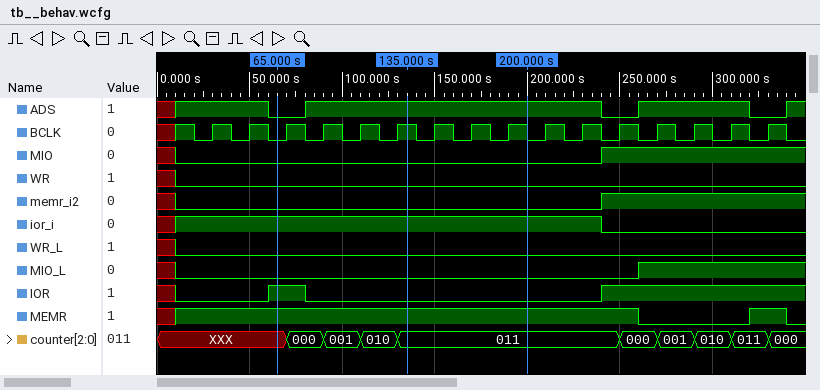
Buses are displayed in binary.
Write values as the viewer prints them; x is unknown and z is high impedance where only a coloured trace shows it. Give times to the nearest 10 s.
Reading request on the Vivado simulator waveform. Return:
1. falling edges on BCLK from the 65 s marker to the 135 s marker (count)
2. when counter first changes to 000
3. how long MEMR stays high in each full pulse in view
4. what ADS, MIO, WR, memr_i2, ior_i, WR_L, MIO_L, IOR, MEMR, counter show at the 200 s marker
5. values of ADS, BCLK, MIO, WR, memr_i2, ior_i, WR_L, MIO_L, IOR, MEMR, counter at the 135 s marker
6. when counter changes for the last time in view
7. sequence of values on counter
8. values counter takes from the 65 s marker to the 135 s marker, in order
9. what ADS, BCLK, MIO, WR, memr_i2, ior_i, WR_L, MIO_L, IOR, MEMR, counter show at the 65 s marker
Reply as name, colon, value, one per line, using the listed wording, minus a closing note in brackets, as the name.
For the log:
falling edges on BCLK from the 65 s marker to the 135 s marker: 3
when counter first changes to 000: 70 s
how long MEMR stays high in each full pulse in view: 20 s
what ADS, MIO, WR, memr_i2, ior_i, WR_L, MIO_L, IOR, MEMR, counter show at the 200 s marker: ADS=1, MIO=0, WR=0, memr_i2=0, ior_i=1, WR_L=0, MIO_L=0, IOR=0, MEMR=1, counter=011
values of ADS, BCLK, MIO, WR, memr_i2, ior_i, WR_L, MIO_L, IOR, MEMR, counter at the 135 s marker: ADS=1, BCLK=1, MIO=0, WR=0, memr_i2=0, ior_i=1, WR_L=0, MIO_L=0, IOR=0, MEMR=1, counter=011
when counter changes for the last time in view: 330 s
sequence of values on counter: XXX, 000, 001, 010, 011, 000, 001, 010, 011, 000
values counter takes from the 65 s marker to the 135 s marker, in order: XXX, 000, 001, 010, 011
what ADS, BCLK, MIO, WR, memr_i2, ior_i, WR_L, MIO_L, IOR, MEMR, counter show at the 65 s marker: ADS=0, BCLK=0, MIO=0, WR=0, memr_i2=0, ior_i=1, WR_L=0, MIO_L=0, IOR=1, MEMR=1, counter=XXX
